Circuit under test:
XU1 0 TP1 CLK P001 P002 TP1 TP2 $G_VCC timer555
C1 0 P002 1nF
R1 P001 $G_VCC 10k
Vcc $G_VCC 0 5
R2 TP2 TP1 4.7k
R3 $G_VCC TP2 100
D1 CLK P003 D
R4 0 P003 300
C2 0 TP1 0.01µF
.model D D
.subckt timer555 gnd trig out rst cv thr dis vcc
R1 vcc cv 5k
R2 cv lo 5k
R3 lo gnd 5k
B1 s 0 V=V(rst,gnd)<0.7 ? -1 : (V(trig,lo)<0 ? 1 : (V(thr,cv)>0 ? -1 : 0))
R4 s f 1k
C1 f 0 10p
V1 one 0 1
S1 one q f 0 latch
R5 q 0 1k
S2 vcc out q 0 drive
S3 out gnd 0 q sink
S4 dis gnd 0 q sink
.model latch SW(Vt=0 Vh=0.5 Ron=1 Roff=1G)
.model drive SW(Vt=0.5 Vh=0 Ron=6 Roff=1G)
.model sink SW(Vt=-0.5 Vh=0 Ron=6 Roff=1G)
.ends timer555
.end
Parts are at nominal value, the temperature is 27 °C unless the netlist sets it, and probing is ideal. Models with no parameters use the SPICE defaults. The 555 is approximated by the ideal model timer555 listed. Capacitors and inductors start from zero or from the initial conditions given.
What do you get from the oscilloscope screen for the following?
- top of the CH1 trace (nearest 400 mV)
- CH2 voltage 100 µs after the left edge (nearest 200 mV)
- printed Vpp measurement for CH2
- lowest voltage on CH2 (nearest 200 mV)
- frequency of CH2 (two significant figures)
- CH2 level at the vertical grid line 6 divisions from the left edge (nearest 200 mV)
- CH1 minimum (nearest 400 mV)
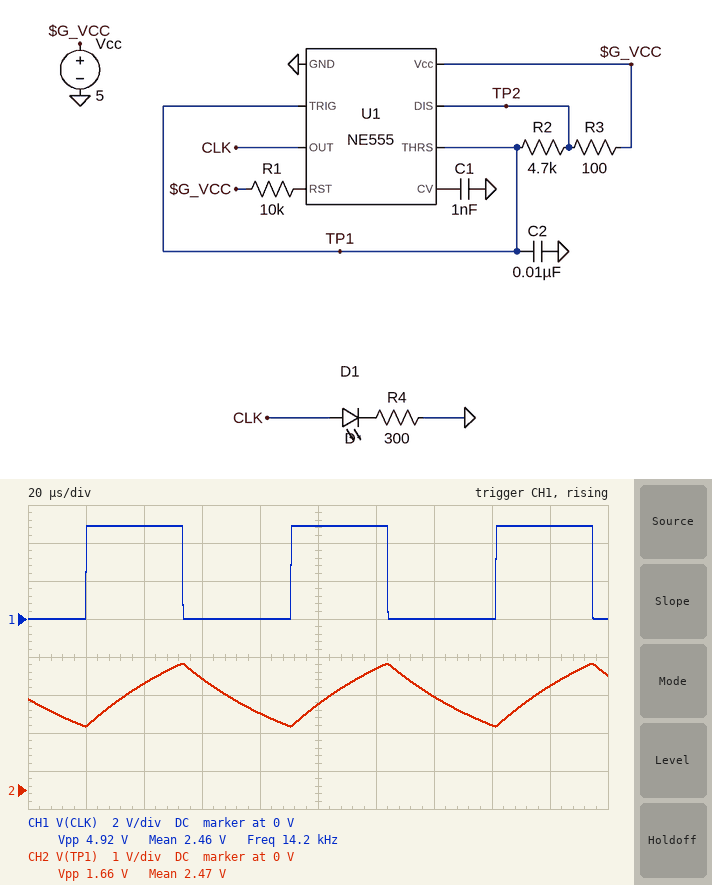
4.8 V
2.2 V
1.66 V
1.6 V
14 kHz
3.2 V
0 V
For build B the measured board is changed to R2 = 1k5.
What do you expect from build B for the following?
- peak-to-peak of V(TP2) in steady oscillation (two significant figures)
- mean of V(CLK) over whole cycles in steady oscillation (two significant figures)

4.6 V
2.4 V
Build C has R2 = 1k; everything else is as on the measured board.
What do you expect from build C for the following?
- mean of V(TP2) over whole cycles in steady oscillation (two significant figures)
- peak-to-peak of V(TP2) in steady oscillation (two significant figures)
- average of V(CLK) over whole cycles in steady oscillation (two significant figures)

2.5 V
4.6 V
2.4 V
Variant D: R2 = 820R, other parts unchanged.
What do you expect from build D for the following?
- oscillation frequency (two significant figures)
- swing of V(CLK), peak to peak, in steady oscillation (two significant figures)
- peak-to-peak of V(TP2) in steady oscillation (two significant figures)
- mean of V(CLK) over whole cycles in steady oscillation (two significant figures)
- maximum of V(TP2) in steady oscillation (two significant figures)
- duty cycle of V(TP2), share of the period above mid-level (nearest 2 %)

78 kHz
4.9 V
4.5 V
2.4 V
4.8 V
50 %
